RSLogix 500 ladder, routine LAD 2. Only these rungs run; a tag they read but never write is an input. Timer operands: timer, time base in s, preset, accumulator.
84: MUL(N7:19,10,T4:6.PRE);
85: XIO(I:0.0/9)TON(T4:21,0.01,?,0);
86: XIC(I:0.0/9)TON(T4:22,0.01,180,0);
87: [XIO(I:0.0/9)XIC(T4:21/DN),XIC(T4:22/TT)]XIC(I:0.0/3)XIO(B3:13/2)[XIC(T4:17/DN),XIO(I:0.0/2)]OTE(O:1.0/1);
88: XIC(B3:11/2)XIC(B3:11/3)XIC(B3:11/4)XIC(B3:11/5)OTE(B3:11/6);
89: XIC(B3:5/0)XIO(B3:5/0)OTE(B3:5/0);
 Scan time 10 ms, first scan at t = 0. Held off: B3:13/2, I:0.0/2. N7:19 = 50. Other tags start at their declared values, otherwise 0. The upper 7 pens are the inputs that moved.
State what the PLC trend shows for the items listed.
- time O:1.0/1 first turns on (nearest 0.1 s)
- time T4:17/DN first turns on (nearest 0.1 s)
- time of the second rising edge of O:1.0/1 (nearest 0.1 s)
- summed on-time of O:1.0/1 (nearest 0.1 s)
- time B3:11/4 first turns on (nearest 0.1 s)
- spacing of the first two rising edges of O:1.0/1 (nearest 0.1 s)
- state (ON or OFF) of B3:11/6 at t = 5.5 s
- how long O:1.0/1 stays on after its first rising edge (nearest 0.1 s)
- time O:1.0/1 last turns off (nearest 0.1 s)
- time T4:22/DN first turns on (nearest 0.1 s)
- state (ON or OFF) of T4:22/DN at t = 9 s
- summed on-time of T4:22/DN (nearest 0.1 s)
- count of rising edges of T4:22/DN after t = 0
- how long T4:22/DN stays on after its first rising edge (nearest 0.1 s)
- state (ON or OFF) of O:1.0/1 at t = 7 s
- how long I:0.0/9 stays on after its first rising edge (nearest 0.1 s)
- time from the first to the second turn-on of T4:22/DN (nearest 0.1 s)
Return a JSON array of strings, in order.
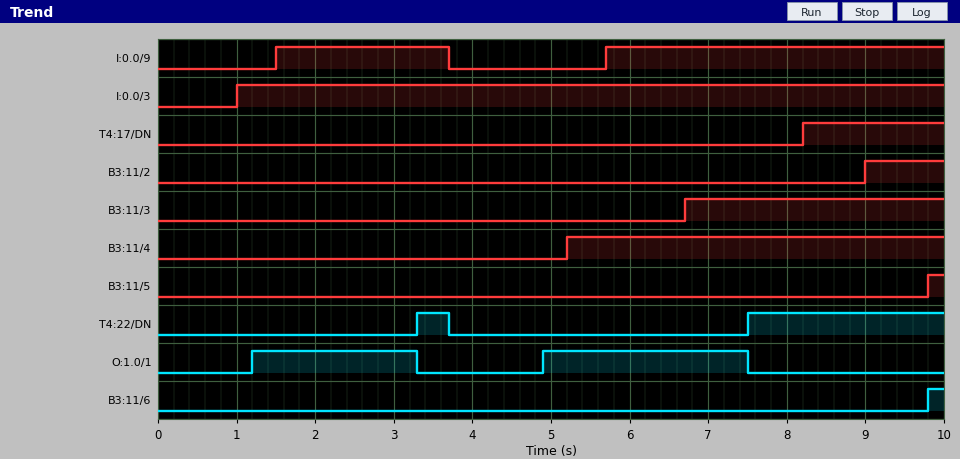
["1.2 s", "8.2 s", "4.9 s", "4.7 s", "5.2 s", "3.7 s", "OFF", "2.1 s", "7.5 s", "3.3 s", "ON", "2.9 s", "2", "0.4 s", "ON", "2.2 s", "4.2 s"]
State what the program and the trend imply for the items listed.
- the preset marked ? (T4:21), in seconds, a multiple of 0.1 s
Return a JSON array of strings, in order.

["1.2 s"]
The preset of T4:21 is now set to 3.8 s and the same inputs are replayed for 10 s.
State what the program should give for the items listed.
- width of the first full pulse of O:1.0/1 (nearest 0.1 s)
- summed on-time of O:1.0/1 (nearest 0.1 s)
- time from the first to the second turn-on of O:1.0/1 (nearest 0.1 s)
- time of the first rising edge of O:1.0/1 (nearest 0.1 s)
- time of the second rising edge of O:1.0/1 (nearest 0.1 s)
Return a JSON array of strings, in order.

["1.8 s", "3.6 s", "4.2 s", "1.5 s", "5.7 s"]
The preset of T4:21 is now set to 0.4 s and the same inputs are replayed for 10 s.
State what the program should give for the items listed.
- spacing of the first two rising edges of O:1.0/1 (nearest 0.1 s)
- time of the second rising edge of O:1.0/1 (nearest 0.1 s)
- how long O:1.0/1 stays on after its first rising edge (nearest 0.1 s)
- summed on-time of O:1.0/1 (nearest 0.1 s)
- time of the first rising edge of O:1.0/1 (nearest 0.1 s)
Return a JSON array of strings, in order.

["3.1 s", "4.1 s", "2.3 s", "5.7 s", "1.0 s"]
